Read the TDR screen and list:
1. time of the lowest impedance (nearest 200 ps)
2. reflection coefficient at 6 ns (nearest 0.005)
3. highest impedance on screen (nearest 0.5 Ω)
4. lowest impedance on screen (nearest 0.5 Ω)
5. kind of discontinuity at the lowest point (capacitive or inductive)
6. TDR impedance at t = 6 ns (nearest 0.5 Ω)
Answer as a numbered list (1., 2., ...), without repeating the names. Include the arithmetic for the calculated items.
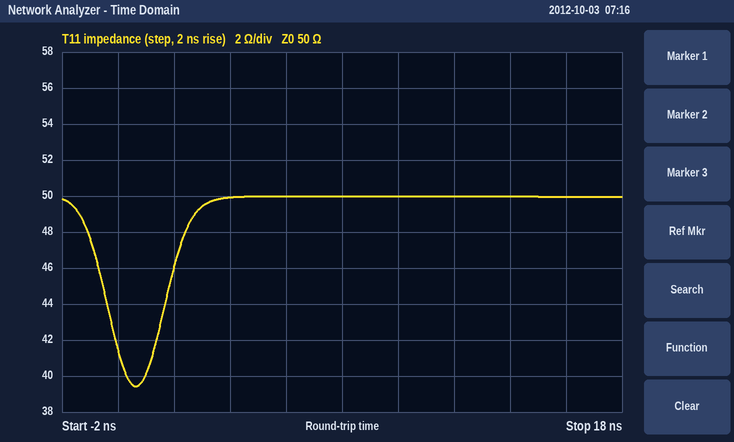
1. 600 ps
2. (50 − 50)/(50 + 50) ≈ 0.000
3. 50.0 Ω
4. 39.5 Ω
5. capacitive
6. 50.0 Ω
